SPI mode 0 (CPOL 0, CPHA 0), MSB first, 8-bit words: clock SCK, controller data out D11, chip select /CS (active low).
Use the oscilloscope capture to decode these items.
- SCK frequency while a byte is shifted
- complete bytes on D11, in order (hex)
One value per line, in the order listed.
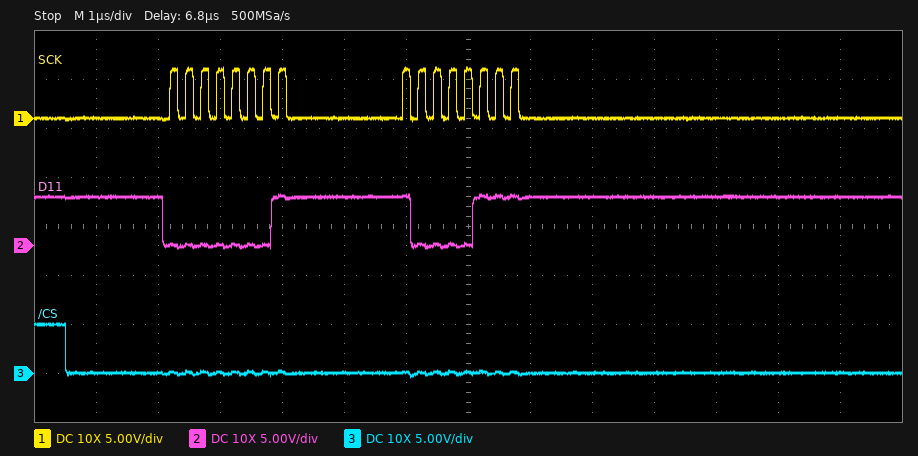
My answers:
4 MHz
01 87
